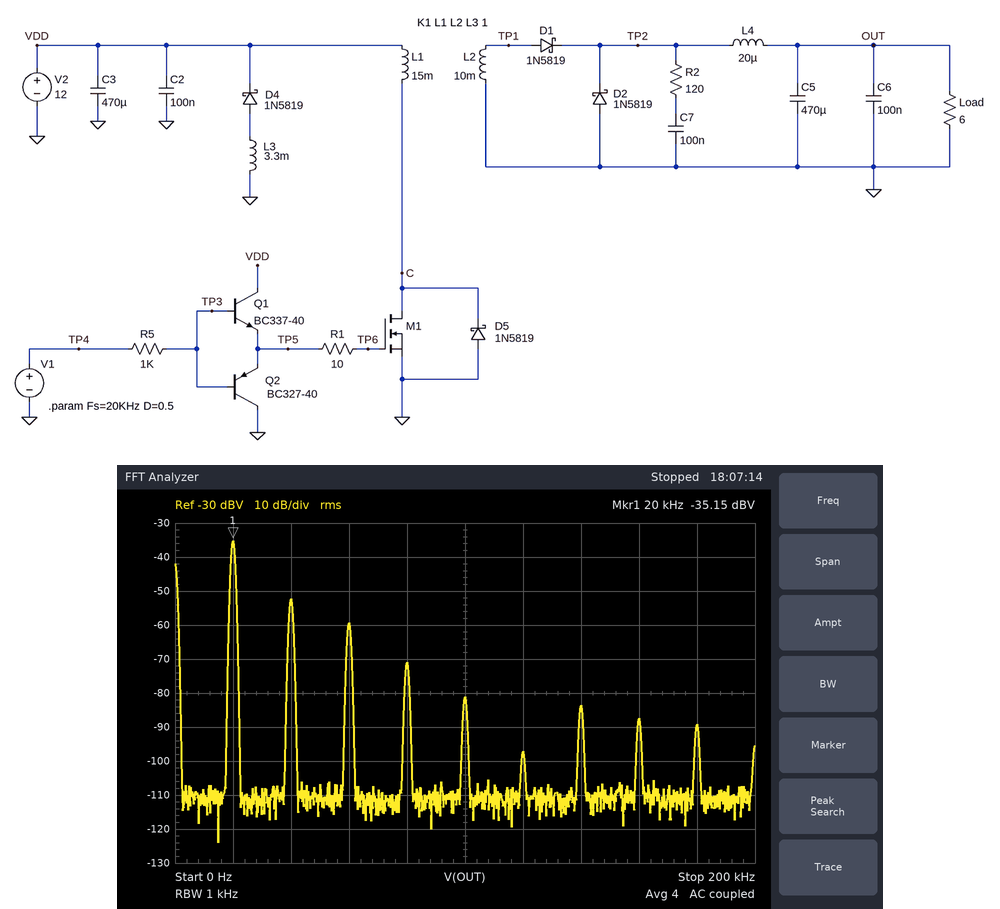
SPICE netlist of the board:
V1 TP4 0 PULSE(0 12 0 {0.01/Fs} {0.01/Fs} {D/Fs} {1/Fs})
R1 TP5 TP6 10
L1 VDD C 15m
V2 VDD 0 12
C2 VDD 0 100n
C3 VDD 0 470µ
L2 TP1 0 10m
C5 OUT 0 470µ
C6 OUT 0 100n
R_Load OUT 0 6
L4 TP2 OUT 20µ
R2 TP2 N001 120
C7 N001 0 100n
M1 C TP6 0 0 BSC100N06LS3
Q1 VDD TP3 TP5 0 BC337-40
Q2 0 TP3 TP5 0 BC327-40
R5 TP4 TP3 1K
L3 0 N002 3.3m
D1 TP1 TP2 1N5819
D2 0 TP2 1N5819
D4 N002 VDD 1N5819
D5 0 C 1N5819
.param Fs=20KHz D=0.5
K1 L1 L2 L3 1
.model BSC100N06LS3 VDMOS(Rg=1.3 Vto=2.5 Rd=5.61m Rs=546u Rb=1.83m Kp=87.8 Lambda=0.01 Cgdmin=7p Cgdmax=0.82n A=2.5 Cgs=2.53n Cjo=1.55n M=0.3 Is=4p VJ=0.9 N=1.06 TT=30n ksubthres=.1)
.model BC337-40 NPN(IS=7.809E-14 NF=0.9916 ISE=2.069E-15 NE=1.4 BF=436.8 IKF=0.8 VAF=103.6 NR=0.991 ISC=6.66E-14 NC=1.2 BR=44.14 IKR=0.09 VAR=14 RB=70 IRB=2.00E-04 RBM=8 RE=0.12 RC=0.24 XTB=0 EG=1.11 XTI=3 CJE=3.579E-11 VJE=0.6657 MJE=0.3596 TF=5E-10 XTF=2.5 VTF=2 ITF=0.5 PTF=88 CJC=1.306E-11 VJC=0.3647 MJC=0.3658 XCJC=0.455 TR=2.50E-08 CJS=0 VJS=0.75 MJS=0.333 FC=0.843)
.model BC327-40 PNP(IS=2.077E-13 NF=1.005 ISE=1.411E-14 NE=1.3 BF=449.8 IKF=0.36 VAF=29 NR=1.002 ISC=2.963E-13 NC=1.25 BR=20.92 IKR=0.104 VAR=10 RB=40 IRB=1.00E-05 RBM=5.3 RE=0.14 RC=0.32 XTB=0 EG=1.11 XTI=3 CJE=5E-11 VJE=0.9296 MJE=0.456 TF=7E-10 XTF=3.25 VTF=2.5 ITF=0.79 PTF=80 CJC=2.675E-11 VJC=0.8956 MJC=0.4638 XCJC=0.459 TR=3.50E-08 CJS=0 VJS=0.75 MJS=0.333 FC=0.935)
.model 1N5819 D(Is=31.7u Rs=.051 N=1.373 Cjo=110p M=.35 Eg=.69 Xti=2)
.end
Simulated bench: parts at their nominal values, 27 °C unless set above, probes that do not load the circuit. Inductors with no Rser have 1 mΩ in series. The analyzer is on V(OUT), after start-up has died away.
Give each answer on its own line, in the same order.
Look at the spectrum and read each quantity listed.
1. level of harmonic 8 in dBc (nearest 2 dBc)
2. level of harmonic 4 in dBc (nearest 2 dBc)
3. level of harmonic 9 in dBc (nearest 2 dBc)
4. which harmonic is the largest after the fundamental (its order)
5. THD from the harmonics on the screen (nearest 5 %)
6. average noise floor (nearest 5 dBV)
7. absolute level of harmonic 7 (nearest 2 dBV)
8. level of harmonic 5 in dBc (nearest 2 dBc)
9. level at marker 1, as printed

-52 dBc
-36 dBc
-54 dBc
2
15 %
-110 dBV
-84 dBV
-46 dBc
-35.15 dBV
